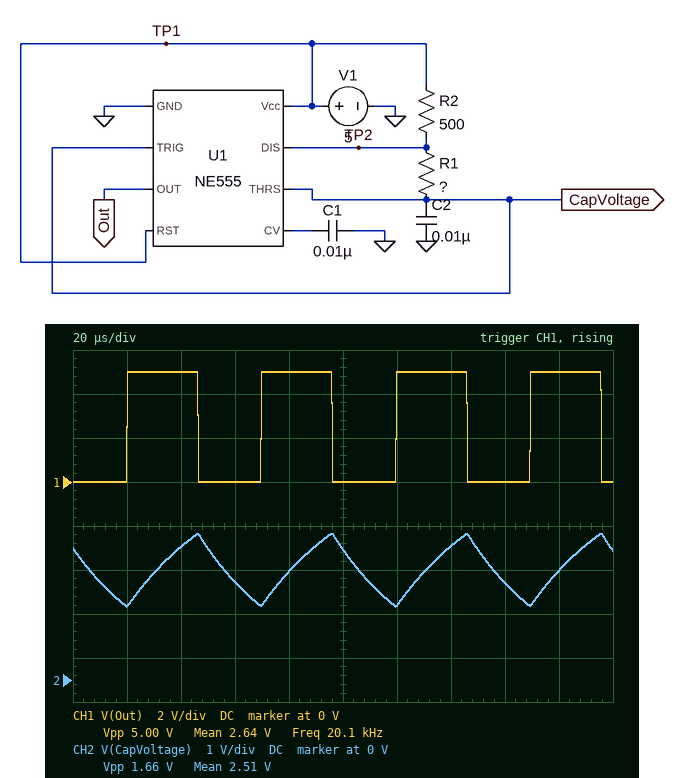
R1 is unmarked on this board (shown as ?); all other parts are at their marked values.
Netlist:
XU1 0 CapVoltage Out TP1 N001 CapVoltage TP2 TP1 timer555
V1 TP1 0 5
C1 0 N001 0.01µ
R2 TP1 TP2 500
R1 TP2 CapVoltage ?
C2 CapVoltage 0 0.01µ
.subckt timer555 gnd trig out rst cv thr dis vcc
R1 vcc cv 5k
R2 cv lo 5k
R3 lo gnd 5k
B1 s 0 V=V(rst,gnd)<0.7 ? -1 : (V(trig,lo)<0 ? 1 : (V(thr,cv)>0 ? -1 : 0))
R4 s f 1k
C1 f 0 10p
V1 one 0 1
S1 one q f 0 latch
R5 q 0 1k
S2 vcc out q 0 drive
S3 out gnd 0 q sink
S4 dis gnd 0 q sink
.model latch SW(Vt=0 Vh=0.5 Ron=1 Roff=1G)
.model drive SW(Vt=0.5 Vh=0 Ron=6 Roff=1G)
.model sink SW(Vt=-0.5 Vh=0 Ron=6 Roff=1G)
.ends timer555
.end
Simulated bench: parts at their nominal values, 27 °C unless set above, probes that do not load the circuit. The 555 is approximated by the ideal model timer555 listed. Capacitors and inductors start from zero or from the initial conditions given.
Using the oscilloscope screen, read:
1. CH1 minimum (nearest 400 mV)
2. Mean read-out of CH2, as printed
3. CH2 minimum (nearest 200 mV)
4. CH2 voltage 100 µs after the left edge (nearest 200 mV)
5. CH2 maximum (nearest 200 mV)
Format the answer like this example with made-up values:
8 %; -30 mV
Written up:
0 V; 2.51 V; 1.6 V; 3.0 V; 3.4 V
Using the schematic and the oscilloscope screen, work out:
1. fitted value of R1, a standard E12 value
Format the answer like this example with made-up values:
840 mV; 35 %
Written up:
3.3 kΩ
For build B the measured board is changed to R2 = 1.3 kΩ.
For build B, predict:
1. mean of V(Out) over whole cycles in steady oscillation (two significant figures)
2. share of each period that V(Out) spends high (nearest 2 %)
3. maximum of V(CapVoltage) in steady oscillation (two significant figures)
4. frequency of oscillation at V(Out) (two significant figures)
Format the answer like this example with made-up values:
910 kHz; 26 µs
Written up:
2.9 V; 58 %; 3.3 V; 18 kHz
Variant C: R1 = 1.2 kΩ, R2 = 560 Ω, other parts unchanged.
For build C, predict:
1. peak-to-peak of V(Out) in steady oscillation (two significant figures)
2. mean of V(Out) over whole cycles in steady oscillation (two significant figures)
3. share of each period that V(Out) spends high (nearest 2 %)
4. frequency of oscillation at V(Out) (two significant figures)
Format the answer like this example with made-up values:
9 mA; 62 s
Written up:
5.0 V; 2.9 V; 58 %; 48 kHz
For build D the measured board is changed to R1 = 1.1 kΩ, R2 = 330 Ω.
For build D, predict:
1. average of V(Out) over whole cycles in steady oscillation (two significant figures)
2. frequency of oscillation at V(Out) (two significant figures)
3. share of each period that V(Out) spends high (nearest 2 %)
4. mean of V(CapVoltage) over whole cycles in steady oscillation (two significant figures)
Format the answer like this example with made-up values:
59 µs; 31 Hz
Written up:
2.8 V; 56 kHz; 56 %; 2.5 V
